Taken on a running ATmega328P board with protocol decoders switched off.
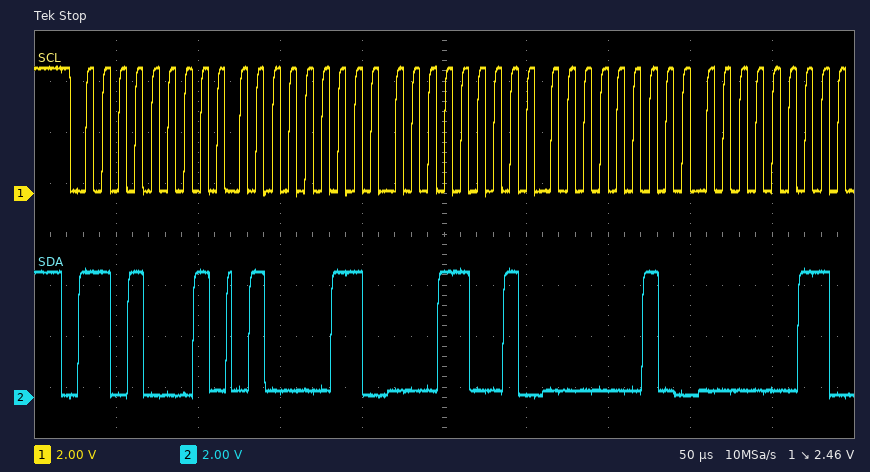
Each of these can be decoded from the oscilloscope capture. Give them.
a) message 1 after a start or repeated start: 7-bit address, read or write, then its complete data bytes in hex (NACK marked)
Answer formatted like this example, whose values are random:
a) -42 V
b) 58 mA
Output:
a) 0x68 read: 43 19 02 03
